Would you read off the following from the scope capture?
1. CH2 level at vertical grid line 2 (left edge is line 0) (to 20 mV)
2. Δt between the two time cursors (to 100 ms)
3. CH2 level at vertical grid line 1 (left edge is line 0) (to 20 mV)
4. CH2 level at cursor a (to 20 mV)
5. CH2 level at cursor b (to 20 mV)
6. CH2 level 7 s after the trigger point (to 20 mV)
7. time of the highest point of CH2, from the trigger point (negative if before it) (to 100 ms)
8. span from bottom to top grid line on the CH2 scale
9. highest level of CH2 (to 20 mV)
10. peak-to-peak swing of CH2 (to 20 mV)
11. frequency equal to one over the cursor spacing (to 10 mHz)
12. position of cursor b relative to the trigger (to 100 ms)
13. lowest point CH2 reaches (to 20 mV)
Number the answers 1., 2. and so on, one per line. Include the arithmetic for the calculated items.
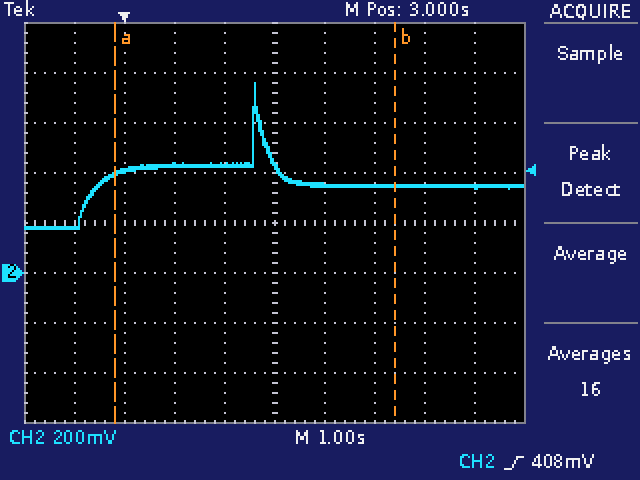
1. 400 mV
2. 5.6 s
3. 180 mV
4. 400 mV
5. 340 mV
6. 340 mV
7. +2.6 s
8. 1.6 V
9. 760 mV
10. 760 mV − (180 mV) = 580 mV
11. 1 / 5.6 s ≈ 180 mHz
12. +5.4 s
13. 180 mV
